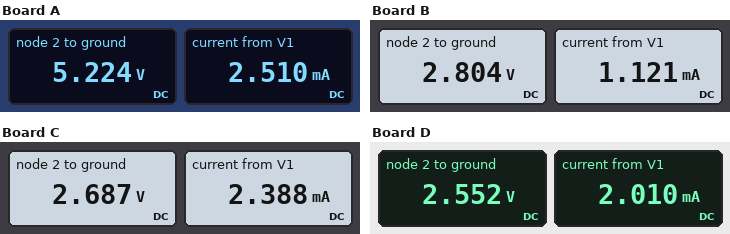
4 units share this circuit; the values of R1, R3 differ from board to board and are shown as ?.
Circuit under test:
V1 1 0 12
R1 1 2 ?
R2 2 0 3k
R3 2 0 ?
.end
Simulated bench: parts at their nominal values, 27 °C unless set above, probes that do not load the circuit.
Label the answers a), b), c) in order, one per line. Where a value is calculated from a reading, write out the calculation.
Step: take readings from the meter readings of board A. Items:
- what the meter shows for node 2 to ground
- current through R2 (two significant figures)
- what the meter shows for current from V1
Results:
a) 5.224 V
b) (5.224 V) / 3 kΩ = 1.7 mA
c) 2.510 mA
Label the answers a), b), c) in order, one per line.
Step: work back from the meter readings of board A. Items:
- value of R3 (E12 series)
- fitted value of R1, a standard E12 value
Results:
a) 6.8 kΩ
b) 2.7 kΩ
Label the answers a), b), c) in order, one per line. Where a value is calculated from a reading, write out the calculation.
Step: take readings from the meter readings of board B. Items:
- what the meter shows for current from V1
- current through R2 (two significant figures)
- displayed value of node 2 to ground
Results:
a) 1.121 mA
b) (2.804 V) / 3 kΩ = 930 µA
c) 2.804 V
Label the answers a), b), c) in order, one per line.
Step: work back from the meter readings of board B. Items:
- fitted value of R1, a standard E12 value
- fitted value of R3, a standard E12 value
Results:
a) 8.2 kΩ
b) 15 kΩ
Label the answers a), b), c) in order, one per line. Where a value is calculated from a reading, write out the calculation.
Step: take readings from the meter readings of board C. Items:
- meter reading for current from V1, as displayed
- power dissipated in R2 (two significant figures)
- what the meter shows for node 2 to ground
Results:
a) 2.388 mA
b) (2.687 V)^2 / 3 kΩ = 2.4 mW
c) 2.687 V
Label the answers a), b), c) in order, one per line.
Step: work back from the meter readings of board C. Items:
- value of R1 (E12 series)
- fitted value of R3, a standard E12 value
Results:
a) 3.9 kΩ
b) 1.8 kΩ
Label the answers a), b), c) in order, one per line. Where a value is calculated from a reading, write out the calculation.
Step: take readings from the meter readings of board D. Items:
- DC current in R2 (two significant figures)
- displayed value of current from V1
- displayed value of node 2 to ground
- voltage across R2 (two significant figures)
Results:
a) (2.552 V) / 3 kΩ = 850 µA
b) 2.010 mA
c) 2.552 V
d) 2.552 V = 2.6 V
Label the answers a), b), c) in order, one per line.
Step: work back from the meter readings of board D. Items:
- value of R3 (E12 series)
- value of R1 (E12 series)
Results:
a) 2.2 kΩ
b) 4.7 kΩ
